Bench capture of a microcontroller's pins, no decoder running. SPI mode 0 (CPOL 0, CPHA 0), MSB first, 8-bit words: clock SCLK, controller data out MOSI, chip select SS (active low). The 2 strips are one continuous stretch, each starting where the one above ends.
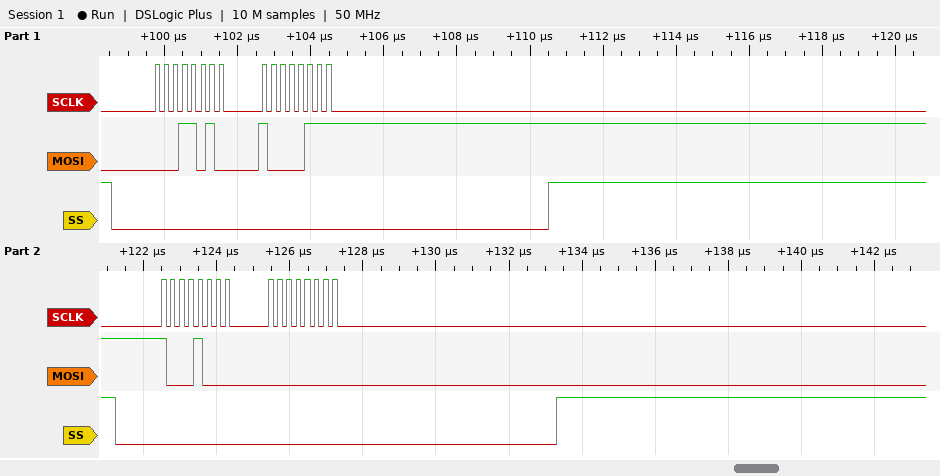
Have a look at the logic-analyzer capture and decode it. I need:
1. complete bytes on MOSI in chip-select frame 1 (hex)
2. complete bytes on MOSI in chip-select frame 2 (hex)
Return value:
1A 87
88 00
